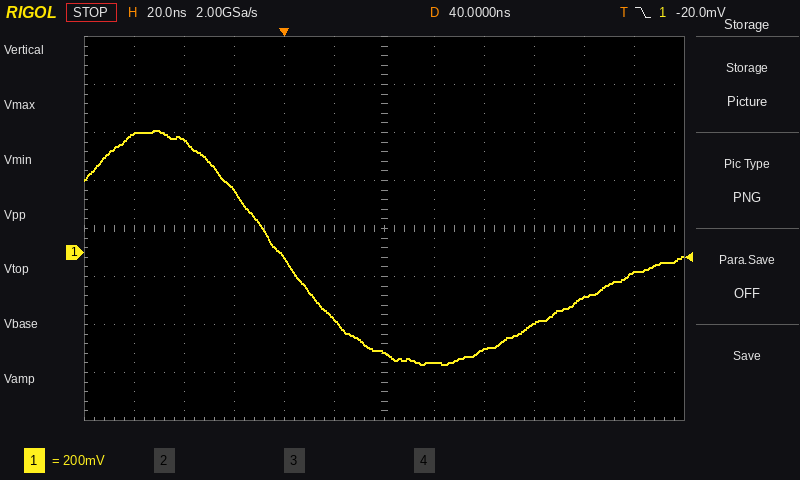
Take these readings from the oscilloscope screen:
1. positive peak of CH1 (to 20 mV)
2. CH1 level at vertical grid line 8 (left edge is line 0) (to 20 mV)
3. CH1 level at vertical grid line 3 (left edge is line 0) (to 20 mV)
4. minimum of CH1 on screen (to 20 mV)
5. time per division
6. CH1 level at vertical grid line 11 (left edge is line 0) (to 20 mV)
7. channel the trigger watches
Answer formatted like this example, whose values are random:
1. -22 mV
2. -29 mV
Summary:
1. 500 mV
2. -400 mV
3. 260 mV
4. -460 mV
5. 20 ns
6. -80 mV
7. CH1
